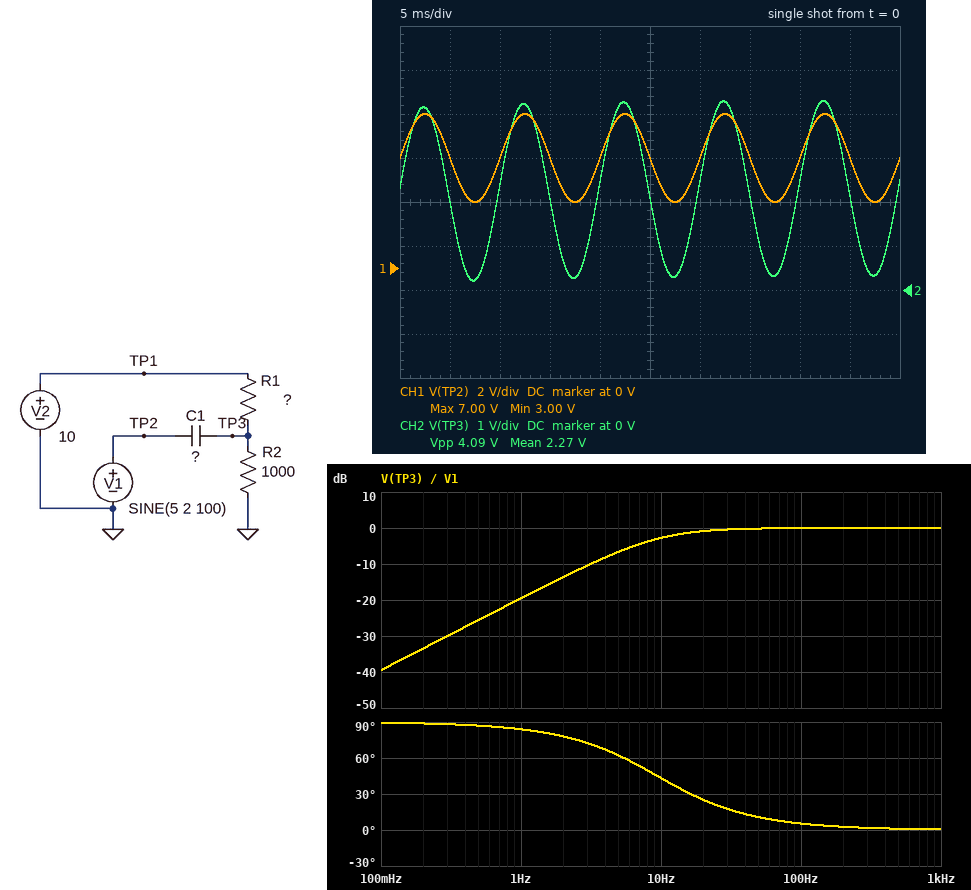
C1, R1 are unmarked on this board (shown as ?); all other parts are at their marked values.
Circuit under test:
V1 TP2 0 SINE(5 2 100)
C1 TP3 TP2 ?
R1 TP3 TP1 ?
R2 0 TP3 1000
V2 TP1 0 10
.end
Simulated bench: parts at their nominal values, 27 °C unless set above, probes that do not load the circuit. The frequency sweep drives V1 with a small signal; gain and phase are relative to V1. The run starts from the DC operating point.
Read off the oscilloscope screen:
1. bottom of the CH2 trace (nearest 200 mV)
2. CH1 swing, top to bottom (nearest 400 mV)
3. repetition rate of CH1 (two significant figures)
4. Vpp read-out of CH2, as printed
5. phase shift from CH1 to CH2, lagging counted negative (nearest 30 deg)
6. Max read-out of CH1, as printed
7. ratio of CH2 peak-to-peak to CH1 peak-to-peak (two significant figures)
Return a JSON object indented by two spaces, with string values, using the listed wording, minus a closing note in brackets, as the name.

{
  "bottom of the CH2 trace": "200 mV",
  "CH1 swing, top to bottom": "4.0 V",
  "repetition rate of CH1": "100 Hz",
  "Vpp read-out of CH2, as printed": "4.09 V",
  "phase shift from CH1 to CH2, lagging counted negative": "0 deg",
  "Max read-out of CH1, as printed": "7.00 V",
  "ratio of CH2 peak-to-peak to CH1 peak-to-peak": "1.0"
}
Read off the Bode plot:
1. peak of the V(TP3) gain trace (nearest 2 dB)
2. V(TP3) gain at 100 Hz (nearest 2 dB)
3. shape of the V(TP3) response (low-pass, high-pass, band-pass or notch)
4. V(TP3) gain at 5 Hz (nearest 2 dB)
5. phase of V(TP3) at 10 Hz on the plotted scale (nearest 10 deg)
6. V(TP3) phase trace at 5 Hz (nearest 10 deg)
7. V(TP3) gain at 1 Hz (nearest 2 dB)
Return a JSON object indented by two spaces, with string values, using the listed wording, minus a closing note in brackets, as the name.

{
  "peak of the V(TP3) gain trace": "0 dB",
  "V(TP3) gain at 100 Hz": "0 dB",
  "shape of the V(TP3) response": "high-pass",
  "V(TP3) gain at 5 Hz": "-6 dB",
  "phase of V(TP3) at 10 Hz on the plotted scale": "40 deg",
  "V(TP3) phase trace at 5 Hz": "60 deg",
  "V(TP3) gain at 1 Hz": "-20 dB"
}
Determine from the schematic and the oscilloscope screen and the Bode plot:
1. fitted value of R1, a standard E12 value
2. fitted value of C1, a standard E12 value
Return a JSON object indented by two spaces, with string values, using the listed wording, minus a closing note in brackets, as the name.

{
  "fitted value of R1, a standard E12 value": "3.3 kΩ",
  "fitted value of C1, a standard E12 value": "22 µF"
}
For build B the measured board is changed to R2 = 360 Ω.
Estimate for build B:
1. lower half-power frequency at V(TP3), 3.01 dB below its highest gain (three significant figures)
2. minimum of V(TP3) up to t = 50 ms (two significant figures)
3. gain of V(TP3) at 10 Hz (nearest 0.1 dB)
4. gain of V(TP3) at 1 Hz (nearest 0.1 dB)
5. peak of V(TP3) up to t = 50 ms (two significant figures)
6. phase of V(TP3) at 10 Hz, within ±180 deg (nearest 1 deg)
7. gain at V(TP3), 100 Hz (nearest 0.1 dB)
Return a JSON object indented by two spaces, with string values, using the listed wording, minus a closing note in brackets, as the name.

{
  "lower half-power frequency at V(TP3), 3.01 dB below its highest gain": "22.3 Hz",
  "minimum of V(TP3) up to t = 50 ms": "-1.1 V",
  "gain of V(TP3) at 10 Hz": "-7.8 dB",
  "gain of V(TP3) at 1 Hz": "-27.0 dB",
  "peak of V(TP3) up to t = 50 ms": "2.9 V",
  "phase of V(TP3) at 10 Hz, within ±180 deg": "66 deg",
  "gain at V(TP3), 100 Hz": "-0.2 dB"
}
